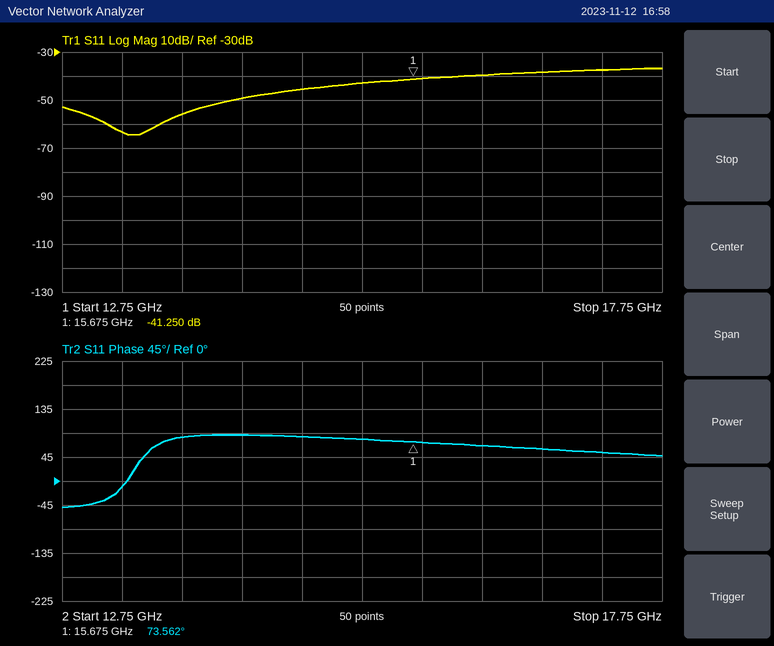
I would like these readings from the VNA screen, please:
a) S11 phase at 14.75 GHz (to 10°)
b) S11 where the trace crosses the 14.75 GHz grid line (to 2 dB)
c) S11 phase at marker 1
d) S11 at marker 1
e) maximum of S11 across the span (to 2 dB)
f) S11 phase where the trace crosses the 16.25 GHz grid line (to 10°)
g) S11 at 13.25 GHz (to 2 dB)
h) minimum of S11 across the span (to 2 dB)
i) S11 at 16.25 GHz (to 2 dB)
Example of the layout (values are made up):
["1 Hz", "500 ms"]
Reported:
["80°", "-46 dB", "73.562°", "-41.250 dB", "-36 dB", "70°", "-64 dB", "-64 dB", "-40 dB"]
